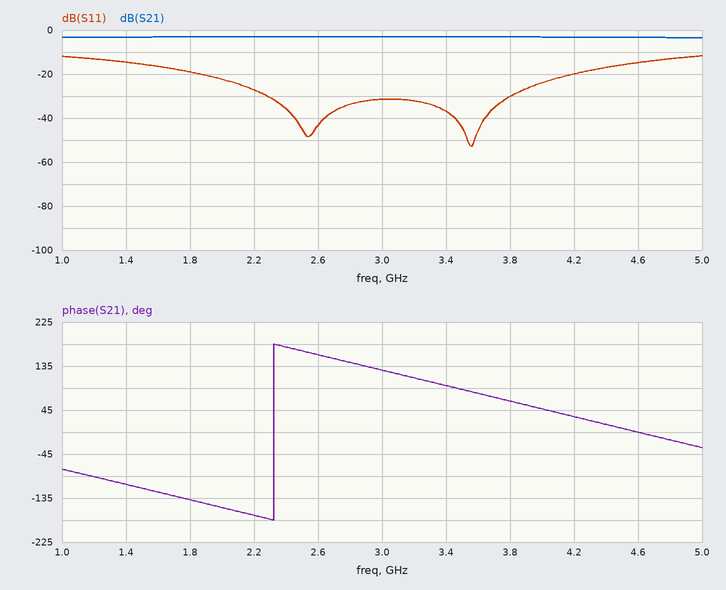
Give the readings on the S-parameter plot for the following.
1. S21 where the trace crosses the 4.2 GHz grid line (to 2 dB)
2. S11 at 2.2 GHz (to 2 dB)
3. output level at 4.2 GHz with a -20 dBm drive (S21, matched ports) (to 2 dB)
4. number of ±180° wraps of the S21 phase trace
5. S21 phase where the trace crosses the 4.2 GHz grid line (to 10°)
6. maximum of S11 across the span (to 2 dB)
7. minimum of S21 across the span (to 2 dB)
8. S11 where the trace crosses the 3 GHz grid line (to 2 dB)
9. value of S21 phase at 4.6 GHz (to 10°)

-4 dB
-28 dB
-24 dBm
1
30°
-12 dB
-4 dB
-32 dB
0°
